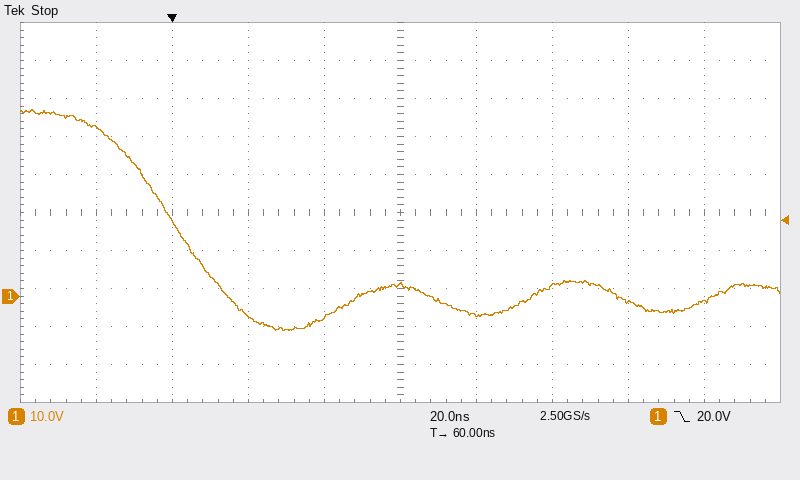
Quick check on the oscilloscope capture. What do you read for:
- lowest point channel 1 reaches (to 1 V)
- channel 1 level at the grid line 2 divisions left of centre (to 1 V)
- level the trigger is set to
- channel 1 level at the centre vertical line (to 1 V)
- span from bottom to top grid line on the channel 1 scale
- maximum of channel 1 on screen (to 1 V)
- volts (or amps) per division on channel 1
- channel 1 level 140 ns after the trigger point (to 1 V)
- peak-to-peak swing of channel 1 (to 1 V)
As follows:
-9 V
-5 V
20.0 V
3 V
100 V
49 V
10 V
-1 V
58 V
